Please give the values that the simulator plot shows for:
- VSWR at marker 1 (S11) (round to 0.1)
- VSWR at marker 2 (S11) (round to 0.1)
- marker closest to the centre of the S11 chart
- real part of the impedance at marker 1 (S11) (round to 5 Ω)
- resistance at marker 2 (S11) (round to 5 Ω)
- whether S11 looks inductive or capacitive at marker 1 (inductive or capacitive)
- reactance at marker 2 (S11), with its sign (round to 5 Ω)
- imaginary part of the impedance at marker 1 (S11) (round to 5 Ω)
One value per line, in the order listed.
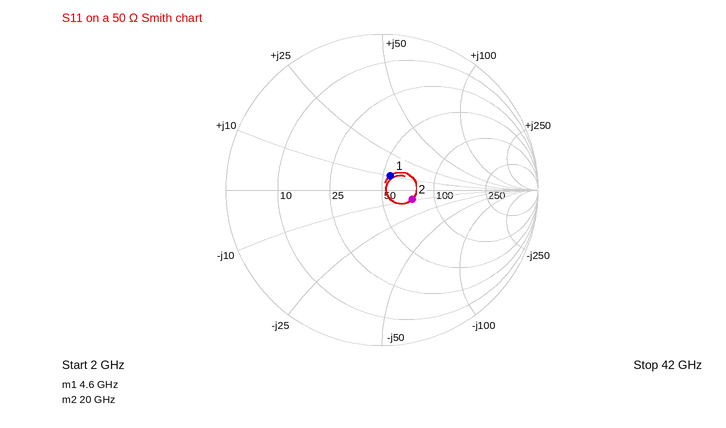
1.2
1.5
marker 1
55 Ω
75 Ω
inductive
-10 Ω
+10 Ω
